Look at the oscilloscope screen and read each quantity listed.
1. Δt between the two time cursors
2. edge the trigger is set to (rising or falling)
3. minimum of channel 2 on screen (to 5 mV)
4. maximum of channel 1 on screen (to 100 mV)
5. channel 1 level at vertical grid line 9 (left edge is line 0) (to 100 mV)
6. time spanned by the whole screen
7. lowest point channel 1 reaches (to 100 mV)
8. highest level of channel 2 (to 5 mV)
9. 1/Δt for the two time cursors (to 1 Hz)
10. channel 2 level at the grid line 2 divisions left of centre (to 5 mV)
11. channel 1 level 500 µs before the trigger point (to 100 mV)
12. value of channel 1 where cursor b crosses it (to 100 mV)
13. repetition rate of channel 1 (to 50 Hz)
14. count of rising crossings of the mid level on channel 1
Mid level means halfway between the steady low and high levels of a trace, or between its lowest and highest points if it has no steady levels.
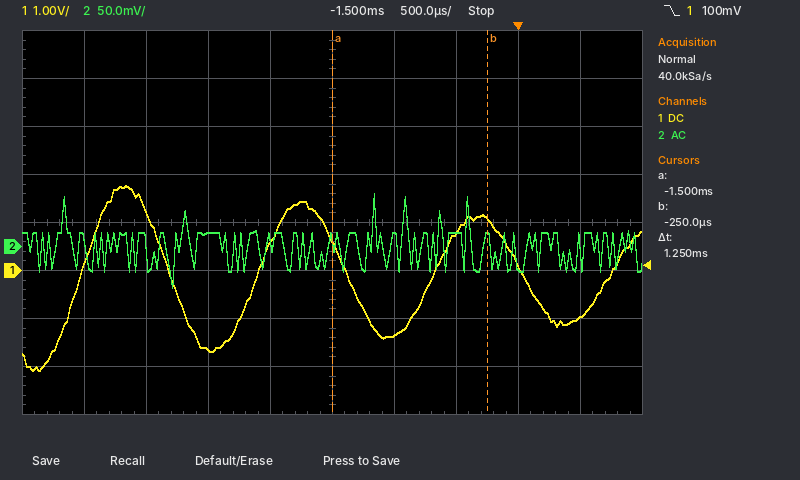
1.25 ms
falling
-45 mV
1.8 V
-1.0 V
5 ms
-2.1 V
55 mV
800 Hz
15 mV
800 mV
1.1 V
700 Hz
4
